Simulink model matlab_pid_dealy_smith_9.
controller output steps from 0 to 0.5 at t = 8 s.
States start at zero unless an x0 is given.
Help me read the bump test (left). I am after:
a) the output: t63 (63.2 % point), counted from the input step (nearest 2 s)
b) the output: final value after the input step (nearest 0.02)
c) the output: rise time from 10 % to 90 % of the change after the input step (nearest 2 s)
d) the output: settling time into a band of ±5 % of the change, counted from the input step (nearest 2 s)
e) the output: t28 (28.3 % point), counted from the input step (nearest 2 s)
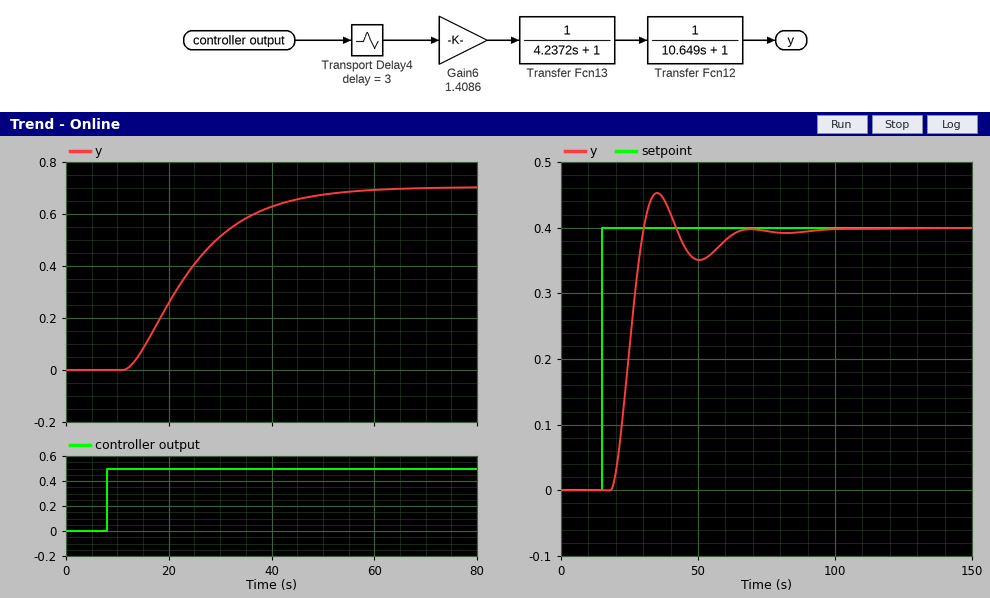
18 s
0.70
26 s
40 s
10 s
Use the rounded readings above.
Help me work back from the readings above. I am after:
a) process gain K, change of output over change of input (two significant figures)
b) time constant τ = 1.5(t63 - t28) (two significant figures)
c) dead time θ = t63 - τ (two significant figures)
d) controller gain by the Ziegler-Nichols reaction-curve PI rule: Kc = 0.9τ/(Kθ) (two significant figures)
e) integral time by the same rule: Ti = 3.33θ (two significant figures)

1.4
12 s
6.0 s
1.3
20 s
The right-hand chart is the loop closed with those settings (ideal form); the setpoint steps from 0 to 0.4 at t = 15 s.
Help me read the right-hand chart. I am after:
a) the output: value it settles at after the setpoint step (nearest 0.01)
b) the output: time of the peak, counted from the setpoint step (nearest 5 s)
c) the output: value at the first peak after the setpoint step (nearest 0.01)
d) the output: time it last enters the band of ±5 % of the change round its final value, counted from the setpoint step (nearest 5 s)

0.40
20 s
0.45
45 s
